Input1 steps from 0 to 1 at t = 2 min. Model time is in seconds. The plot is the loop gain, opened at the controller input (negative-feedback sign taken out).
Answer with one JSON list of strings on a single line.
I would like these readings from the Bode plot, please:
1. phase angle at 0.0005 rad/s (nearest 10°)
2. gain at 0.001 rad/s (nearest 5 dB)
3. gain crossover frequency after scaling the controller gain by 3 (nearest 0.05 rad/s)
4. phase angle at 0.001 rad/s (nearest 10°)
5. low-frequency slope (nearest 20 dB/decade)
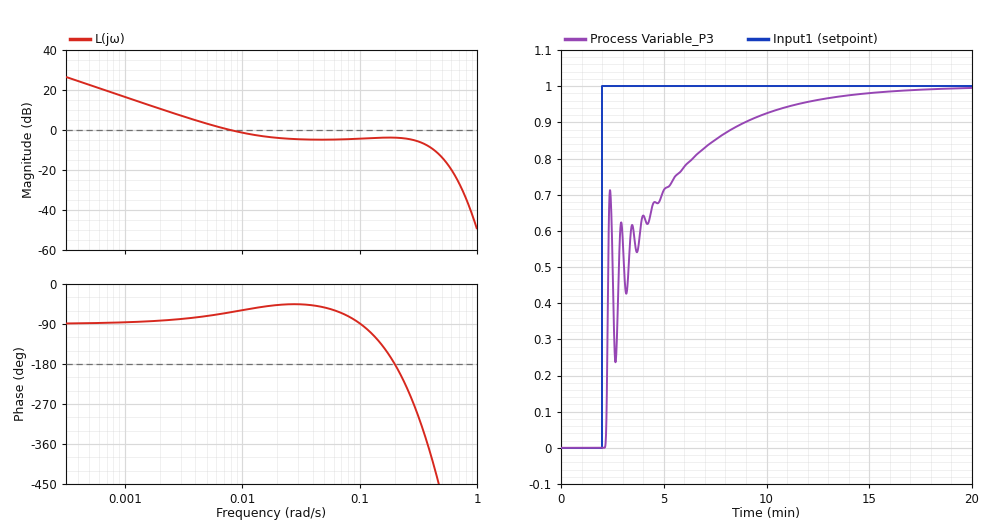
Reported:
["-90°", "15 dB", "0.40 rad/s", "-90°", "-20 dB/decade"]
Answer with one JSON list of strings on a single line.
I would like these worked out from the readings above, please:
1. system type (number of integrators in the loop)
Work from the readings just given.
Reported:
["1"]
